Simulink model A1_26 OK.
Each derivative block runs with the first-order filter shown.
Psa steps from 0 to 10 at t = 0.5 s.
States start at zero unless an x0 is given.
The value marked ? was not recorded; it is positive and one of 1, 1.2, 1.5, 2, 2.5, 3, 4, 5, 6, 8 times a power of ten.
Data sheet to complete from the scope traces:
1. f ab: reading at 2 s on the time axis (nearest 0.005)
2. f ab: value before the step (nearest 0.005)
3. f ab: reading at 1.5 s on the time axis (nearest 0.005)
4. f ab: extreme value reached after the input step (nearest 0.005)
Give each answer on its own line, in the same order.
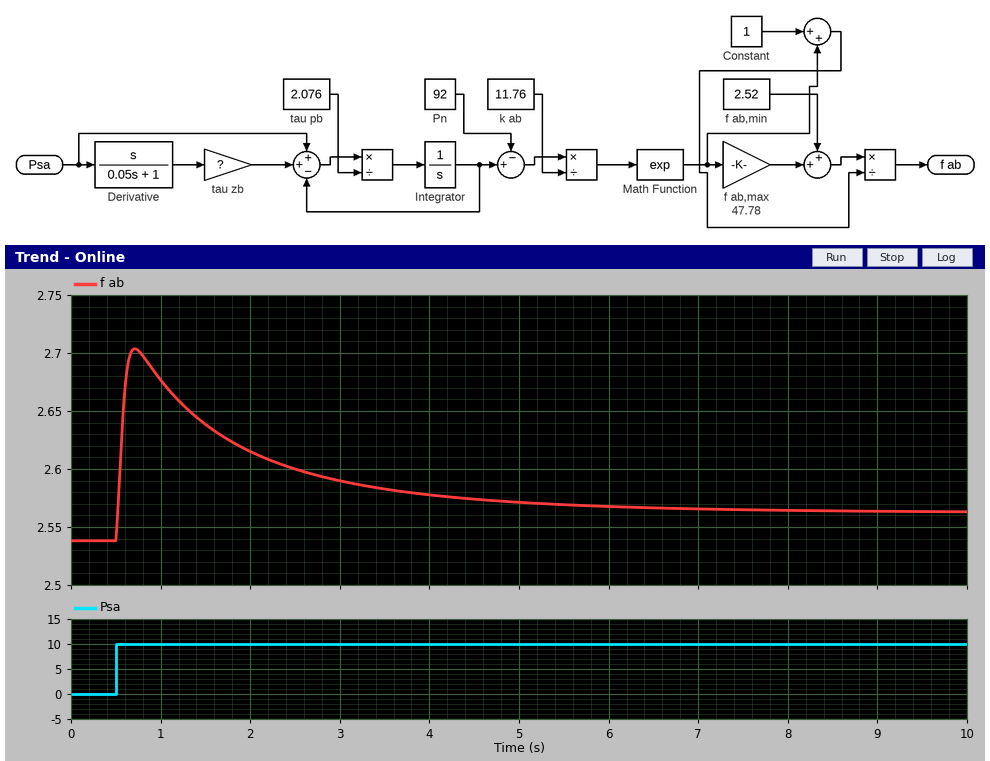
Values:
2.615
2.540
2.640
2.705
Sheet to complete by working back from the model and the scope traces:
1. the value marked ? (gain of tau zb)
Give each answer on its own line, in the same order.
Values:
6
